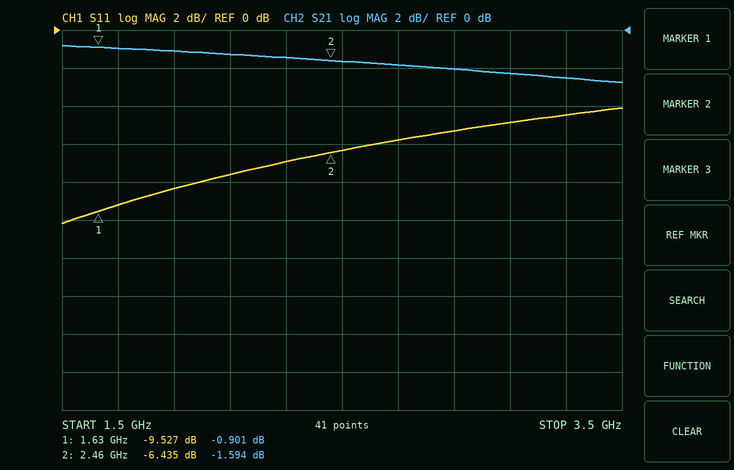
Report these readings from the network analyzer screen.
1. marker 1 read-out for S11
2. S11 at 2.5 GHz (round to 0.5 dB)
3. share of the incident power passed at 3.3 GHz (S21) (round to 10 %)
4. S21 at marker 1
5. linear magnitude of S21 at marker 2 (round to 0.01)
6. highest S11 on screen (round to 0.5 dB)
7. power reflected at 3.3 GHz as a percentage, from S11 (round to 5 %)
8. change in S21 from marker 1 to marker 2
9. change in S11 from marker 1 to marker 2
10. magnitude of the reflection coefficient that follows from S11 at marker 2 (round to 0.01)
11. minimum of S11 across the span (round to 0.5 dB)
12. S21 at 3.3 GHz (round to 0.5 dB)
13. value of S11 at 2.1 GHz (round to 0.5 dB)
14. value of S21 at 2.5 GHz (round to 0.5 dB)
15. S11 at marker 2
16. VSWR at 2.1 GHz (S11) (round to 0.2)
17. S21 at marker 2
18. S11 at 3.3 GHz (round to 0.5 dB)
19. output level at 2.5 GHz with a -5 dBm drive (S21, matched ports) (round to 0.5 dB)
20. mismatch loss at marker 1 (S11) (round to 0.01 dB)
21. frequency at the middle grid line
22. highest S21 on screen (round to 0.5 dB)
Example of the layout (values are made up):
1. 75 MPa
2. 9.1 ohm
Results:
1. -9.527 dB
2. -6.5 dB
3. 60 %
4. -0.901 dB
5. 0.83
6. -4.0 dB
7. 35 %
8. -0.693 dB
9. 3.092 dB
10. 0.48
11. -10.0 dB
12. -2.5 dB
13. -7.5 dB
14. -1.5 dB
15. -6.435 dB
16. 2.4
17. -1.594 dB
18. -4.5 dB
19. -6.5 dBm
20. 0.51 dB
21. 2.5 GHz
22. -1.0 dB
